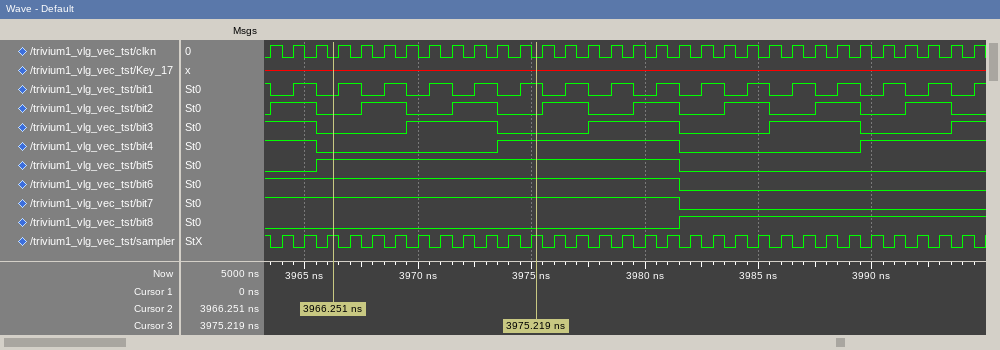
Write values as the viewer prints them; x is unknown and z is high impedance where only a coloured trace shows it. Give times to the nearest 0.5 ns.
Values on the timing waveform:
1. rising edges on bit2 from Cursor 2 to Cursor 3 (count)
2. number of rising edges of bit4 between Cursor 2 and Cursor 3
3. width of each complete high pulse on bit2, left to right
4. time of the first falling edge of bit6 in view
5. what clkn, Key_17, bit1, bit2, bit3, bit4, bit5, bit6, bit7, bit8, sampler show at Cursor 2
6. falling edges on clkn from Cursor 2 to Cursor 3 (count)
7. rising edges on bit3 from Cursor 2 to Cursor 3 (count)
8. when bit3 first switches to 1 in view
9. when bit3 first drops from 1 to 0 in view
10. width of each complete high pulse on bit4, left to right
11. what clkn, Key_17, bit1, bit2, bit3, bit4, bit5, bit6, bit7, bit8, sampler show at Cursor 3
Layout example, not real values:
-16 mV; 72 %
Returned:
2; 1; 2 ns, 2 ns, 2 ns, 2 ns, 2 ns, 2 ns, 2 ns, 2 ns; 3981.5 ns; clkn=0, Key_17=x, bit1=0, bit2=0, bit3=0, bit4=0, bit5=1, bit6=1, bit7=1, bit8=0, sampler=1; 9; 1; 3969.5 ns; 3965.5 ns; 8 ns; clkn=0, Key_17=x, bit1=1, bit2=0, bit3=0, bit4=1, bit5=1, bit6=1, bit7=1, bit8=0, sampler=1
